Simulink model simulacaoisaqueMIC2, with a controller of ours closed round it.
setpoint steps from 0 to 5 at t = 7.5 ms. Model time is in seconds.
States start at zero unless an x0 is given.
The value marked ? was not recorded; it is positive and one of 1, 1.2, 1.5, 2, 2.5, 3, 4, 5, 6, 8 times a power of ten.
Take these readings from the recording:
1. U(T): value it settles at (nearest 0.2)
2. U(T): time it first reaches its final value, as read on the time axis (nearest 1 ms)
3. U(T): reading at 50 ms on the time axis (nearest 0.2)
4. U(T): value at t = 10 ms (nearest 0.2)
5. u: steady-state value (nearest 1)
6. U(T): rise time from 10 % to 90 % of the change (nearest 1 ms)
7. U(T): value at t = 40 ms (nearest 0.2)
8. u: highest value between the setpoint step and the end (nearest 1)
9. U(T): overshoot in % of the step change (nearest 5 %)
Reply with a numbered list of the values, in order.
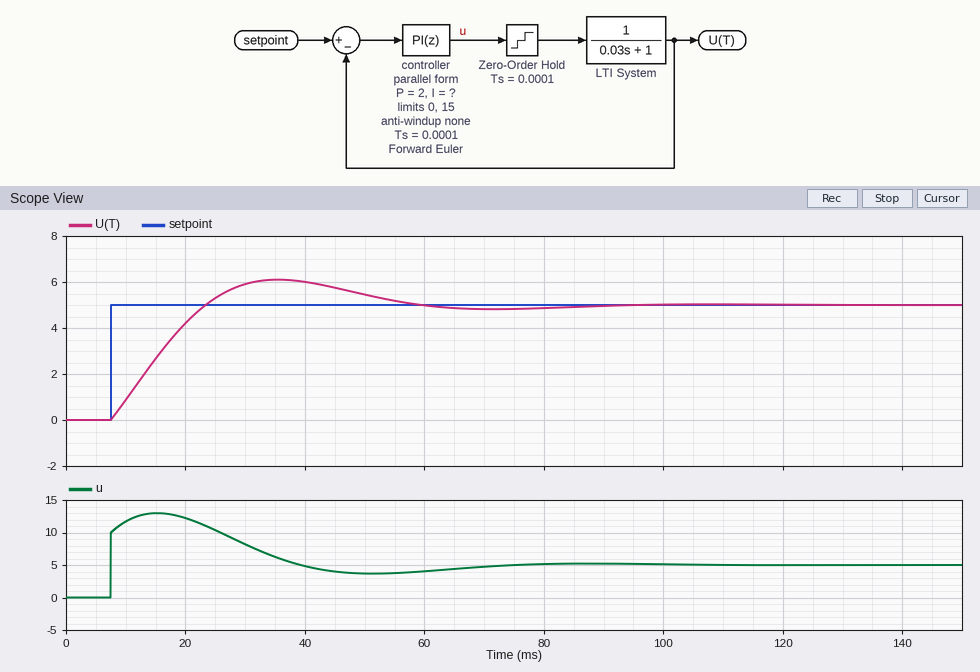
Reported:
1. 5.0
2. 23 ms
3. 5.4
4. 0.8
5. 5
6. 12 ms
7. 6.0
8. 13
9. 20 %
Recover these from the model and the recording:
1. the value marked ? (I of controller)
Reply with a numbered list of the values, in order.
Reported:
1. 300
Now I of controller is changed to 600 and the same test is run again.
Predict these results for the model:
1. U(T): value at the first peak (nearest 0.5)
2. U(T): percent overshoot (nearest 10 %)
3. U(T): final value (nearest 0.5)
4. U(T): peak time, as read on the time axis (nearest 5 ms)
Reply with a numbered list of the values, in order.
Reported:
1. 7.0
2. 40 %
3. 5.0
4. 30 ms
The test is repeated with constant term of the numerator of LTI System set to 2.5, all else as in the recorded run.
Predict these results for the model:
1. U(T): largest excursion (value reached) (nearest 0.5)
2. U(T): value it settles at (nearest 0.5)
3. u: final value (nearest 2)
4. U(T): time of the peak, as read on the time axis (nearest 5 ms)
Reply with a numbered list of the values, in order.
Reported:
1. 6.0
2. 5.0
3. 2
4. 25 ms
